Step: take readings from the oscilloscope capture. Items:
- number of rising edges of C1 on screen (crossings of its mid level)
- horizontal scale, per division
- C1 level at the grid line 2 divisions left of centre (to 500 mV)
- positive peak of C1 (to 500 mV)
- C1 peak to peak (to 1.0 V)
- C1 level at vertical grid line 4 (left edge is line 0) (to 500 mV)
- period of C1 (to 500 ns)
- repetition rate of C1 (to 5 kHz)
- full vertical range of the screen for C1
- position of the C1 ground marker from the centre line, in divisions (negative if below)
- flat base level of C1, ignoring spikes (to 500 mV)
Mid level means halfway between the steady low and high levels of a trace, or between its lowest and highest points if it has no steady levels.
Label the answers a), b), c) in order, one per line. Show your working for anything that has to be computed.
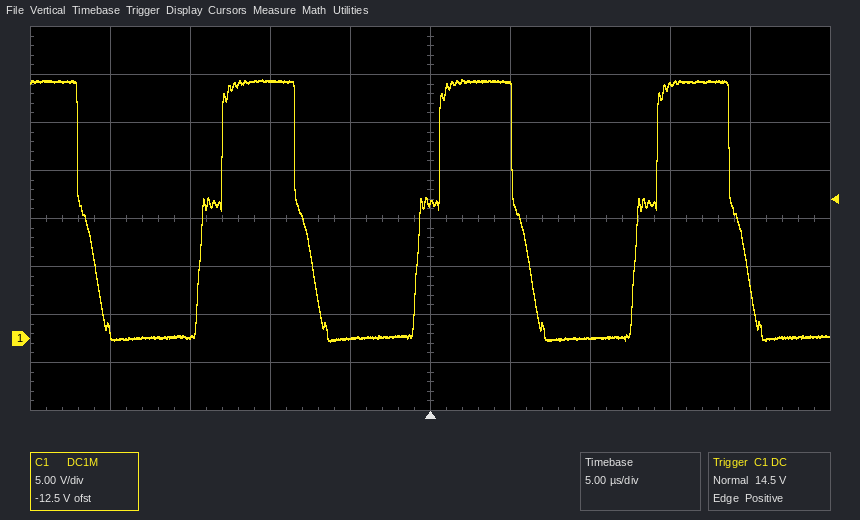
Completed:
a) 3
b) 5 µs
c) 27.0 V
d) 27.0 V
e) 27.0 V
f) 0.0 V
g) 13.5 µs
h) 1 / 13.5 µs ≈ 74.1 kHz, so 75 kHz to the nearest 5 kHz
i) 40 V
j) -2.5 div
k) 0.0 V
